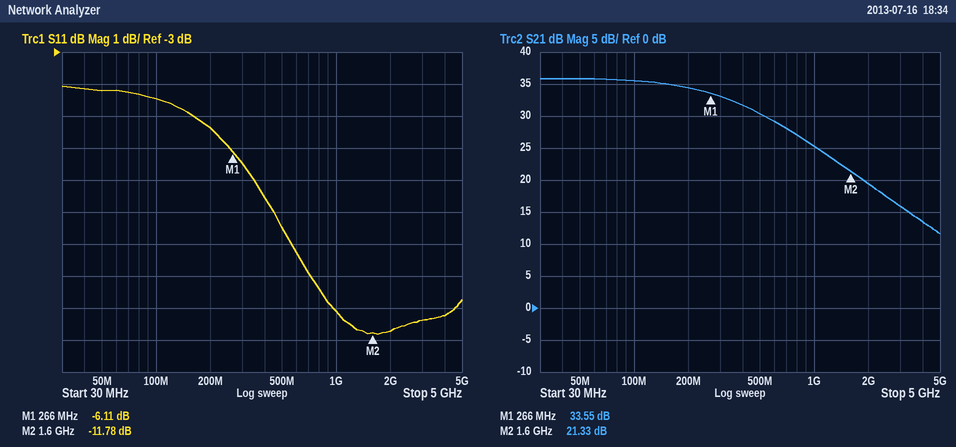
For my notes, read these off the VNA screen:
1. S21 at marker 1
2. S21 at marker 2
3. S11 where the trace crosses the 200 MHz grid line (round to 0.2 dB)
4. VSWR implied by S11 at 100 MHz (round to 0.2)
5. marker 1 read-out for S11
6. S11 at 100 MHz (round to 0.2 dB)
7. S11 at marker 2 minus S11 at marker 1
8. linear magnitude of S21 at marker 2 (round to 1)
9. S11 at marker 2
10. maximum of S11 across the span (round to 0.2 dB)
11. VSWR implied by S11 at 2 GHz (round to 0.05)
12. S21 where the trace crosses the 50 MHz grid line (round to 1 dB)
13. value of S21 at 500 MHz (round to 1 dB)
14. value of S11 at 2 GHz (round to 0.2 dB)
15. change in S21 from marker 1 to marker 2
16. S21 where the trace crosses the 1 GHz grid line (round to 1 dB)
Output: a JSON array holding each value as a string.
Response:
["33.55 dB", "21.33 dB", "-5.4 dB", "4.0", "-6.11 dB", "-4.4 dB", "-5.67 dB", "12", "-11.78 dB", "-4.0 dB", "1.70", "36 dB", "30 dB", "-11.8 dB", "-12.22 dB", "25 dB"]
